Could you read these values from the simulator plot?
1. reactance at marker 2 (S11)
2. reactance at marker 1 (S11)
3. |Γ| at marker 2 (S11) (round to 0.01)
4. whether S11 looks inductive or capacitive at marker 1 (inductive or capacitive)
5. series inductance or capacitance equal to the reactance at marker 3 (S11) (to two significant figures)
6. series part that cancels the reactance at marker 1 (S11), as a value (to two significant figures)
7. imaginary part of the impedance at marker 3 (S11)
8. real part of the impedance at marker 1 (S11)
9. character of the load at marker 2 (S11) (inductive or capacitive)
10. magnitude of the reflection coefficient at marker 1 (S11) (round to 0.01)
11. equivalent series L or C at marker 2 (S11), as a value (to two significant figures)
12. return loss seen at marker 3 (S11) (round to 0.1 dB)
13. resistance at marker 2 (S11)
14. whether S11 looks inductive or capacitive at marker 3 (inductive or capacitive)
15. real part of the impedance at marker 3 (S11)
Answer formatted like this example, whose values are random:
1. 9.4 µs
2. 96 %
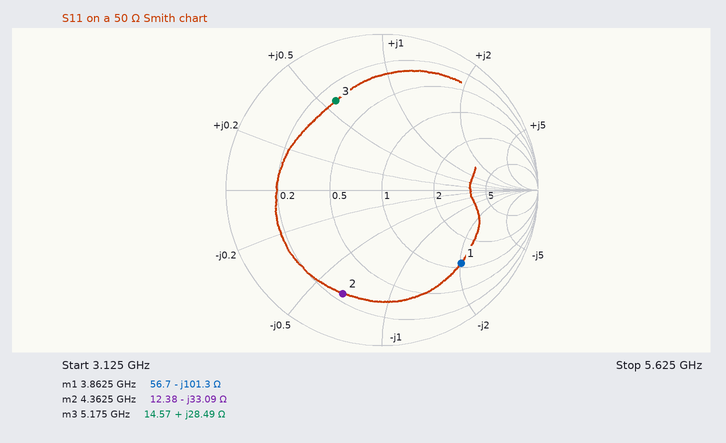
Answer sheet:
1. -33.09 Ω
2. -101.3 Ω
3. 0.71
4. capacitive
5. 880 pH
6. 4.2 nH
7. +28.49 Ω
8. 56.7 Ω
9. capacitive
10. 0.69
11. 1.1 pF
12. 3.8 dB
13. 12.38 Ω
14. inductive
15. 14.57 Ω
